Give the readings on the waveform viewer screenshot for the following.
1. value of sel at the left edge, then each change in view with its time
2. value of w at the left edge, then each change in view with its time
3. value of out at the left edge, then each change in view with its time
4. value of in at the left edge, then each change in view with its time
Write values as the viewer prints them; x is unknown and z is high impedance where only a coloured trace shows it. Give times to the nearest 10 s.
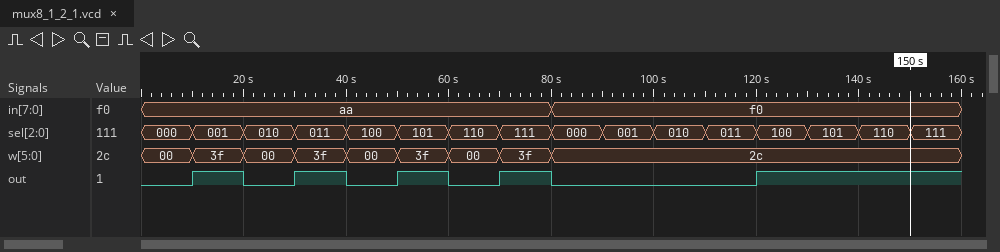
000, 001 at 10 s, 010 at 20 s, 011 at 30 s, 100 at 40 s, 101 at 50 s, 110 at 60 s, 111 at 70 s, 000 at 80 s, 001 at 90 s, 010 at 100 s, 011 at 110 s, 100 at 120 s, 101 at 130 s, 110 at 140 s, 111 at 150 s
00, 3f at 10 s, 00 at 20 s, 3f at 30 s, 00 at 40 s, 3f at 50 s, 00 at 60 s, 3f at 70 s, 2c at 80 s
0, 1 at 10 s, 0 at 20 s, 1 at 30 s, 0 at 40 s, 1 at 50 s, 0 at 60 s, 1 at 70 s, 0 at 80 s, 1 at 120 s
aa, f0 at 80 s
